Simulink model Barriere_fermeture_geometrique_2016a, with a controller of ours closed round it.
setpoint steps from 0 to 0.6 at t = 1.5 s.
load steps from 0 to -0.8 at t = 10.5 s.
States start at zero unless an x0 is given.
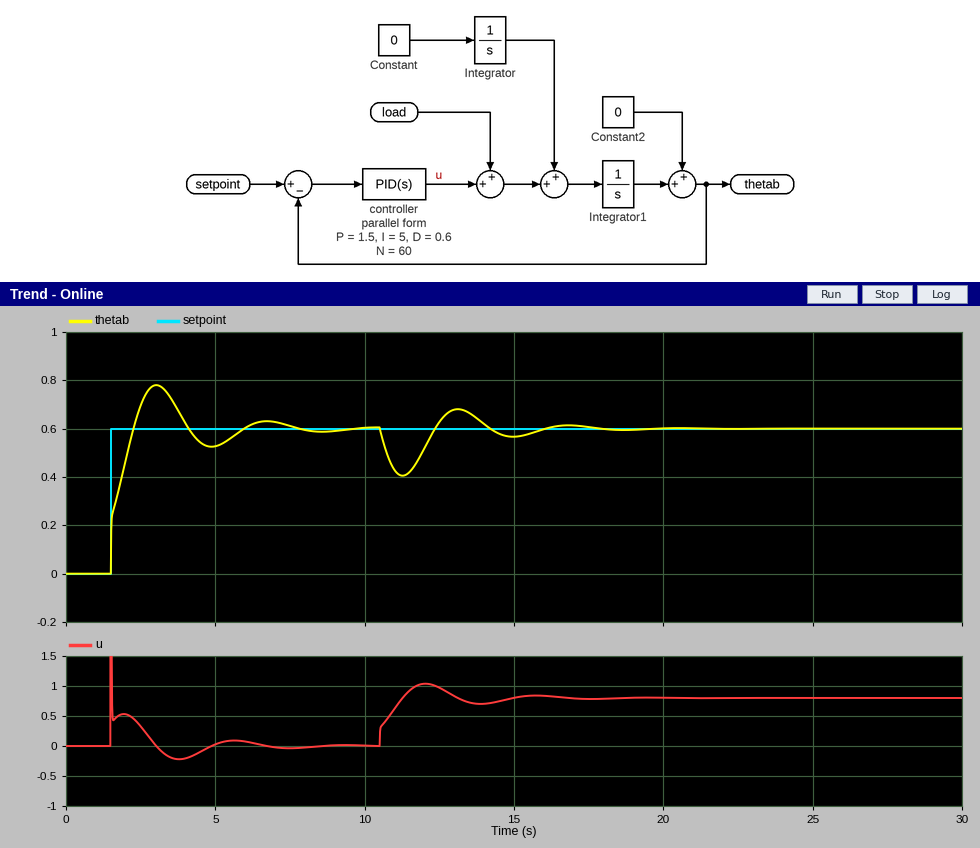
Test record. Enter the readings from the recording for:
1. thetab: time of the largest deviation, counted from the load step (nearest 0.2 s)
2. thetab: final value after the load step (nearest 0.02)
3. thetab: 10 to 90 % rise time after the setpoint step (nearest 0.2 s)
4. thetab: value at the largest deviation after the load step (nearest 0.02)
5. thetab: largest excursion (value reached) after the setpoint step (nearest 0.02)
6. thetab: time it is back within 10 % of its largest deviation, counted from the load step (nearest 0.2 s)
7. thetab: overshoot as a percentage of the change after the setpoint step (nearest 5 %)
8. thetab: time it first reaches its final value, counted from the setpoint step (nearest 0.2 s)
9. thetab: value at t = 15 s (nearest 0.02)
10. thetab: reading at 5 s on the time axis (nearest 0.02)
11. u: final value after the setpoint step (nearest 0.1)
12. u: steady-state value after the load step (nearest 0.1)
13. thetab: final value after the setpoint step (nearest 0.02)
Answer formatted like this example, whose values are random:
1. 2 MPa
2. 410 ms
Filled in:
1. 0.8 s
2. 0.60
3. 0.6 s
4. 0.40
5. 0.78
6. 5.0 s
7. 30 %
8. 0.8 s
9. 0.56
10. 0.52
11. 0.0
12. 0.8
13. 0.60
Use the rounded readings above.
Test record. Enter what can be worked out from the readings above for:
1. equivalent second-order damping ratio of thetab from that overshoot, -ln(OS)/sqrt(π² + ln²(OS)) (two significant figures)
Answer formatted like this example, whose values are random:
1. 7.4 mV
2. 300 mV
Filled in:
1. 0.36
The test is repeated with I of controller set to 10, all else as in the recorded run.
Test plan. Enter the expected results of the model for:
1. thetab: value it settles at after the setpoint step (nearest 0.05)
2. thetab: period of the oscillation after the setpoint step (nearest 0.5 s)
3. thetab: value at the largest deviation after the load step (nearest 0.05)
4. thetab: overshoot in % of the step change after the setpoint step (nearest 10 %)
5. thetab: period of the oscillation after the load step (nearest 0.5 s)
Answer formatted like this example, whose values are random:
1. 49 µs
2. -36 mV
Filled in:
1. 0.60
2. 2.5 s
3. 0.45
4. 40 %
5. 2.5 s
